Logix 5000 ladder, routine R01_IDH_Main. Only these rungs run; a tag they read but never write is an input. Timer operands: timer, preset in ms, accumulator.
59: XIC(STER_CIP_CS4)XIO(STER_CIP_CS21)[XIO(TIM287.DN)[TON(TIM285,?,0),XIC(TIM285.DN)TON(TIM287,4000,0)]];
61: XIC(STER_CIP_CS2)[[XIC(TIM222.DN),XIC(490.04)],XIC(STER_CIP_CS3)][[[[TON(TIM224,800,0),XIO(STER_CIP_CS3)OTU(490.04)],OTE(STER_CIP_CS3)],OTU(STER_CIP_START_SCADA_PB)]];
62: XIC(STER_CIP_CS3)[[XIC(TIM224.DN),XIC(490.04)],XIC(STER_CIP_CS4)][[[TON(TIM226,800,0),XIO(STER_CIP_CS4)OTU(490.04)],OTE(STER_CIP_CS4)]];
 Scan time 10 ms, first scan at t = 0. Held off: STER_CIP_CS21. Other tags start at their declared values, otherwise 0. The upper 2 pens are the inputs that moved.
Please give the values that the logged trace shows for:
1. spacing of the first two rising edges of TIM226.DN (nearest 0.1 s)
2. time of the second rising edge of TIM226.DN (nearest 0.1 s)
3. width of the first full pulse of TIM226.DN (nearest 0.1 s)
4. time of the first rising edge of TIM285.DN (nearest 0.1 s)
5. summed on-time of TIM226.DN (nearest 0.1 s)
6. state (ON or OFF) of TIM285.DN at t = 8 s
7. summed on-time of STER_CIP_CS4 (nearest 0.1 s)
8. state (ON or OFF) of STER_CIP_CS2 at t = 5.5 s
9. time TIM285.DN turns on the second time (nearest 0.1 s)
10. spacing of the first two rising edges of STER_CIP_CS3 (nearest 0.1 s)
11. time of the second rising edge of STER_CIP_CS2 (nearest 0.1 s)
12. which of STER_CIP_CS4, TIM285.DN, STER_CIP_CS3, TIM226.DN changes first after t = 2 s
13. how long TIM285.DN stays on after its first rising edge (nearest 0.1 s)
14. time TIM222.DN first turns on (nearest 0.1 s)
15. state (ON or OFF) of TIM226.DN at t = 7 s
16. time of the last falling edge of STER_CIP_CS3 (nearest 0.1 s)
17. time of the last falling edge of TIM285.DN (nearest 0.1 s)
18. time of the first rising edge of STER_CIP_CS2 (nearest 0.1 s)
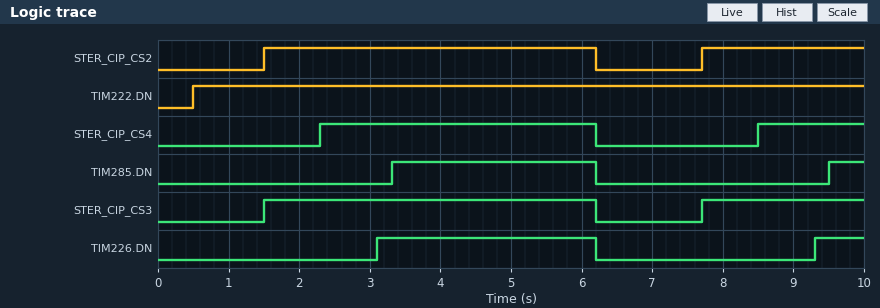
6.2 s
9.3 s
3.1 s
3.3 s
3.8 s
OFF
5.4 s
ON
9.5 s
6.2 s
7.7 s
STER_CIP_CS4
2.9 s
0.5 s
OFF
6.2 s
6.2 s
1.5 s
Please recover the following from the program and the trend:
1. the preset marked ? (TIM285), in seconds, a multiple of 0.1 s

1.0 s
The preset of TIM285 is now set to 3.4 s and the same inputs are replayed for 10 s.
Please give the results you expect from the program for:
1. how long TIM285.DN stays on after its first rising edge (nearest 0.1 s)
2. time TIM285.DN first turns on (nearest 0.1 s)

0.5 s
5.7 s
